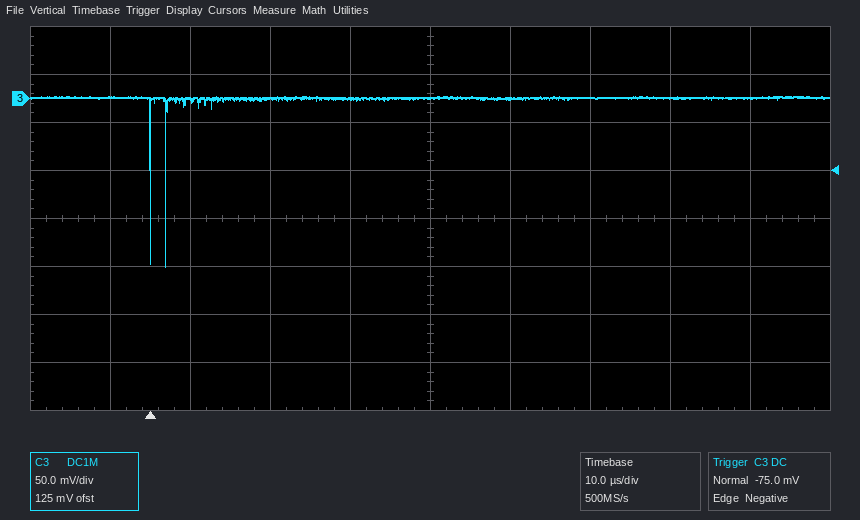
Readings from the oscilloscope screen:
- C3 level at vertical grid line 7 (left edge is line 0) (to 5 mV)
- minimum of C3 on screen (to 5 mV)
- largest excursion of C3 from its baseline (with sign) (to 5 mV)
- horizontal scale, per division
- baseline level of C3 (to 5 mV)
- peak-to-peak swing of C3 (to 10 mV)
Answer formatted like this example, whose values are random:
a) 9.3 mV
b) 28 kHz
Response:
a) 0 mV
b) -175 mV
c) -175 mV
d) 10 µs
e) 0 mV
f) 180 mV
